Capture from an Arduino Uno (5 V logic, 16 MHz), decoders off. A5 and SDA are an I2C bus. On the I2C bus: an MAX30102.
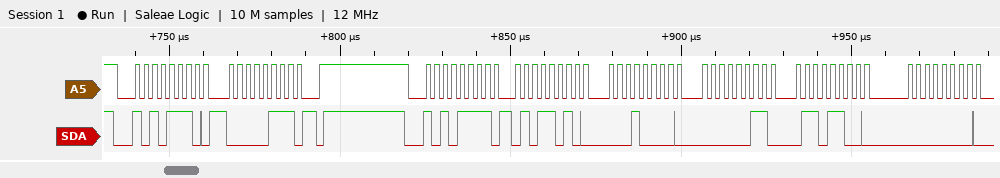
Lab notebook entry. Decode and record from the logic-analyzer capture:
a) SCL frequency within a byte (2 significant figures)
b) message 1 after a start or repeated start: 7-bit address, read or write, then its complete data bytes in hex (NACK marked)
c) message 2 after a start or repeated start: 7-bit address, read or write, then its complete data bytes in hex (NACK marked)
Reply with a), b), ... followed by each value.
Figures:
a) 400 kHz
b) 0x57 write: 07
c) 0x57 read: 5A 10 03 6C 00
